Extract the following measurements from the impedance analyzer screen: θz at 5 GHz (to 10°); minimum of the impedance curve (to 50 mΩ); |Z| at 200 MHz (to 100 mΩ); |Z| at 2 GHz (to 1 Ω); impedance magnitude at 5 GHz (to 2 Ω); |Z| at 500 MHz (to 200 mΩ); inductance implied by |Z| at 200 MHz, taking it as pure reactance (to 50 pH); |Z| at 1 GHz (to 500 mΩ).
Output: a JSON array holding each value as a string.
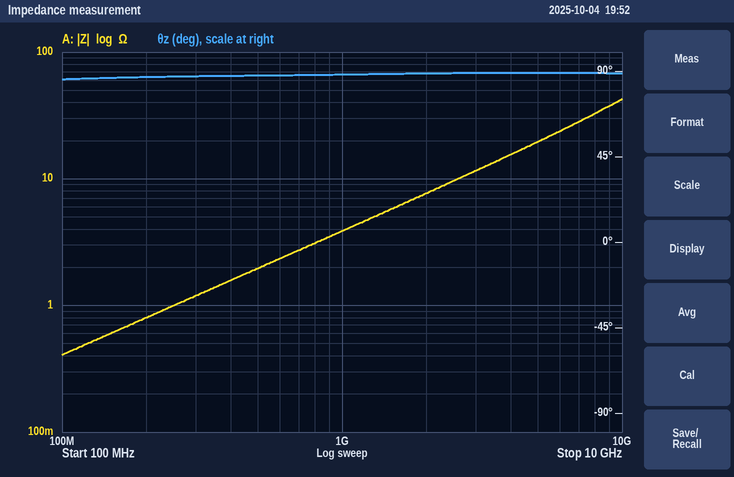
["90°", "400 mΩ", "800 mΩ", "8 Ω", "20 Ω", "2.0 Ω", "650 pH", "4.0 Ω"]
